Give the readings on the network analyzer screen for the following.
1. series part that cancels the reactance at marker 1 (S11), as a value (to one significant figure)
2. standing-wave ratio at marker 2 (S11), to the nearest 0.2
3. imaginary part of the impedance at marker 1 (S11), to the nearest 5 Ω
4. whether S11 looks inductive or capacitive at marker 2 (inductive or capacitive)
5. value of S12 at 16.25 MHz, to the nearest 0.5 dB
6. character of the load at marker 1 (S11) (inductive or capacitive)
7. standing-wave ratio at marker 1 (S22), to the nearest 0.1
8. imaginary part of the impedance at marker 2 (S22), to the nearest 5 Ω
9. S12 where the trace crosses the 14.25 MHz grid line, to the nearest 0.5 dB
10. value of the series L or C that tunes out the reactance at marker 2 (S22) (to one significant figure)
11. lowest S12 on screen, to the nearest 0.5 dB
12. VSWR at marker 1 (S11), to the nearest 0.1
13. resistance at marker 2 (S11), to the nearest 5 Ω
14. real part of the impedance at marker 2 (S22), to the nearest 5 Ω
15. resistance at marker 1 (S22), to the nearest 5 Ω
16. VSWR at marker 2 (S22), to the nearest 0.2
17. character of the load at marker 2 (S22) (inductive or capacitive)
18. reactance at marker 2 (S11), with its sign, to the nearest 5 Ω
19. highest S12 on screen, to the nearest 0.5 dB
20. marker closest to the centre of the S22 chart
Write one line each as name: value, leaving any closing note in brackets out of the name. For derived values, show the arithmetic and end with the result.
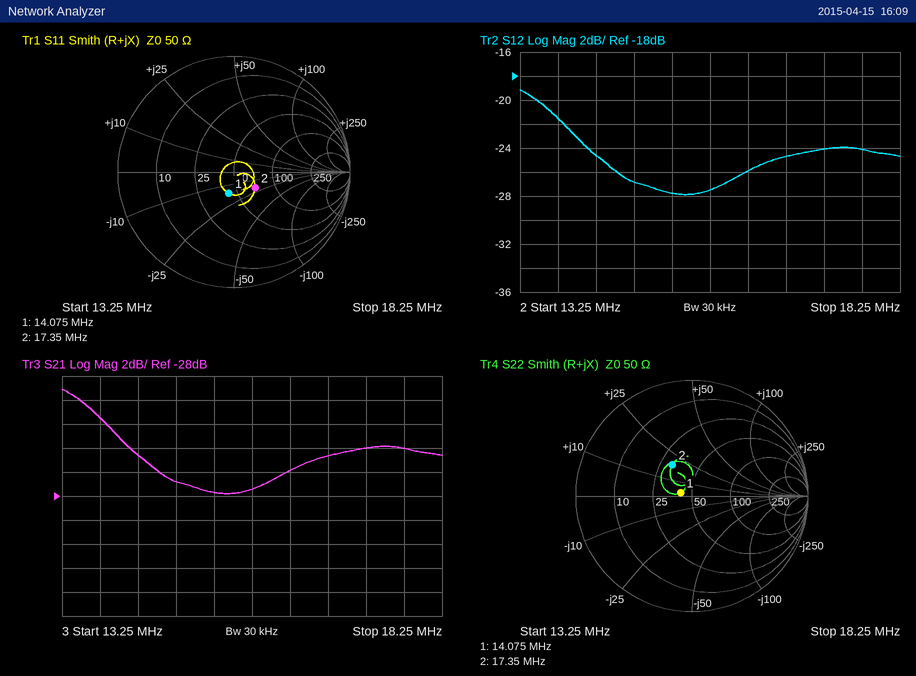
series part that cancels the reactance at marker 1 (S11), as a value: L = 15 Ω/(2π × 14.075 MHz) ≈ 170 nH, so 200 nH to one significant figure
standing-wave ratio at marker 2 (S11), to the nearest 0.2: 1.6
imaginary part of the impedance at marker 1 (S11), to the nearest 5 Ω: -15 Ω
whether S11 looks inductive or capacitive at marker 2: capacitive
value of S12 at 16.25 MHz, to the nearest 0.5 dB: -26.0 dB
character of the load at marker 1 (S11): capacitive
standing-wave ratio at marker 1 (S22), to the nearest 0.1: 1.2
imaginary part of the impedance at marker 2 (S22), to the nearest 5 Ω: +20 Ω
S12 where the trace crosses the 14.25 MHz grid line, to the nearest 0.5 dB: -24.5 dB
value of the series L or C that tunes out the reactance at marker 2 (S22): C = 1/(2π × 17.35 MHz × 20 Ω) ≈ 459 pF, so 500 pF to one significant figure
lowest S12 on screen, to the nearest 0.5 dB: -28.0 dB
VSWR at marker 1 (S11), to the nearest 0.1: 1.5
resistance at marker 2 (S11), to the nearest 5 Ω: 70 Ω
real part of the impedance at marker 2 (S22), to the nearest 5 Ω: 30 Ω
resistance at marker 1 (S22), to the nearest 5 Ω: 40 Ω
VSWR at marker 2 (S22), to the nearest 0.2: 2.0
character of the load at marker 2 (S22): inductive
reactance at marker 2 (S11), with its sign, to the nearest 5 Ω: -20 Ω
highest S12 on screen, to the nearest 0.5 dB: -19.0 dB
marker closest to the centre of the S22 chart: marker 1
